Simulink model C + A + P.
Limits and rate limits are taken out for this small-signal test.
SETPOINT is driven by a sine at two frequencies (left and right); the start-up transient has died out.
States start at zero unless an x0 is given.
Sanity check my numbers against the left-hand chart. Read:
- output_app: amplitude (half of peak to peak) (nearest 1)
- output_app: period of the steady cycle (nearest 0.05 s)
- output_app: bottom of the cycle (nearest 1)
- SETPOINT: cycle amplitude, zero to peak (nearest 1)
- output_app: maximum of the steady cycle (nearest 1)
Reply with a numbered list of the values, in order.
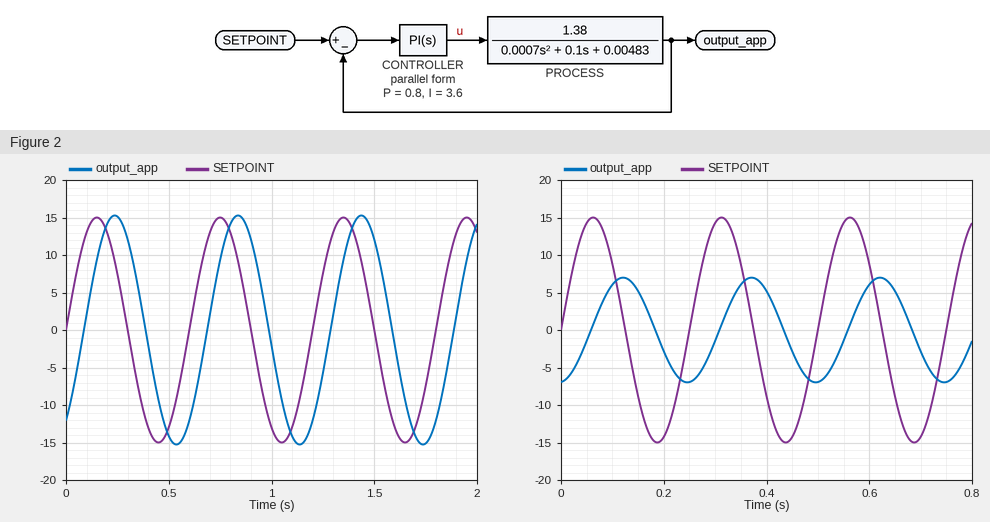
1. 15
2. 0.60 s
3. -15
4. 15
5. 15
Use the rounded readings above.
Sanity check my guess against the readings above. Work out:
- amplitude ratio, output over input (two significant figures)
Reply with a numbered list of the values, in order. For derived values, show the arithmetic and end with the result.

1. 15 / 15 = 1.0
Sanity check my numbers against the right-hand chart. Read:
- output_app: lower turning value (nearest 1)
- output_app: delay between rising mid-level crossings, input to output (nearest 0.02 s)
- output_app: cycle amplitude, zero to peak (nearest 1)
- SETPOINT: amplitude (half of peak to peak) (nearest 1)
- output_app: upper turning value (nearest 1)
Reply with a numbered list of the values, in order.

1. -7
2. 0.06 s
3. 7
4. 15
5. 7
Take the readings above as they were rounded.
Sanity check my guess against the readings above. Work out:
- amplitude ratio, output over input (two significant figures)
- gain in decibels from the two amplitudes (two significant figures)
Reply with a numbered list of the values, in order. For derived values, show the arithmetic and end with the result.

1. 7 / 15 = 0.47
2. 20 log10(7 / 15) = -6.6 dB
